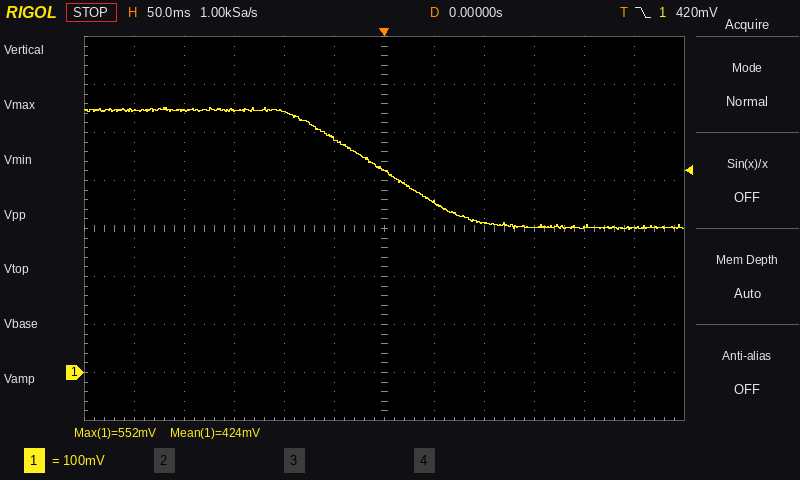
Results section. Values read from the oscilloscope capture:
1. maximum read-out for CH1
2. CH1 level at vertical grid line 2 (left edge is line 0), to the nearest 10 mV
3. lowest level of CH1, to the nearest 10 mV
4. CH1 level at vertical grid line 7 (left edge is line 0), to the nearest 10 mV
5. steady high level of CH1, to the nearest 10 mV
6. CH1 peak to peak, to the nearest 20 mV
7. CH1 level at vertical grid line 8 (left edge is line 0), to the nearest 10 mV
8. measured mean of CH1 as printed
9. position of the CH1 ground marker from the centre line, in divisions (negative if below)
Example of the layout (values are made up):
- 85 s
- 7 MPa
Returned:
- 552 mV
- 550 mV
- 300 mV
- 350 mV
- 550 mV
- 260 mV
- 310 mV
- 424 mV
- -3.0 div
